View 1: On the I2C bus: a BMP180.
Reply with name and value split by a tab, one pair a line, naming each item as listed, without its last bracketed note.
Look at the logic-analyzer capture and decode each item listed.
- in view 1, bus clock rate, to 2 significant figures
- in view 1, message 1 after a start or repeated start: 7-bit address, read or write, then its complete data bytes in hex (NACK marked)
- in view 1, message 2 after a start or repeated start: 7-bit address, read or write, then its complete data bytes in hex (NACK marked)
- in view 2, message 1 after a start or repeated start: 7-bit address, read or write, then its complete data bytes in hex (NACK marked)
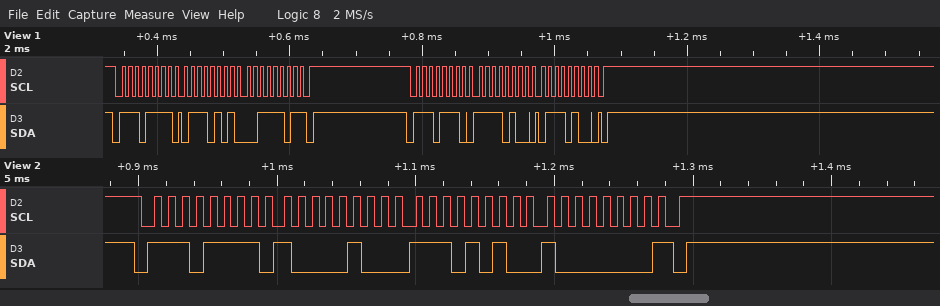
in view 1, bus clock rate, to 2 significant figures	100 kHz
in view 1, message 1 after a start or repeated start: 7-bit address, read or write, then its complete data bytes in hex	0x77 read: 75 3D NACK
in view 1, message 2 after a start or repeated start: 7-bit address, read or write, then its complete data bytes in hex	0x77 write: F4 74
in view 2, message 1 after a start or repeated start: 7-bit address, read or write, then its complete data bytes in hex	0x77 read: 84 EA 80 NACK
